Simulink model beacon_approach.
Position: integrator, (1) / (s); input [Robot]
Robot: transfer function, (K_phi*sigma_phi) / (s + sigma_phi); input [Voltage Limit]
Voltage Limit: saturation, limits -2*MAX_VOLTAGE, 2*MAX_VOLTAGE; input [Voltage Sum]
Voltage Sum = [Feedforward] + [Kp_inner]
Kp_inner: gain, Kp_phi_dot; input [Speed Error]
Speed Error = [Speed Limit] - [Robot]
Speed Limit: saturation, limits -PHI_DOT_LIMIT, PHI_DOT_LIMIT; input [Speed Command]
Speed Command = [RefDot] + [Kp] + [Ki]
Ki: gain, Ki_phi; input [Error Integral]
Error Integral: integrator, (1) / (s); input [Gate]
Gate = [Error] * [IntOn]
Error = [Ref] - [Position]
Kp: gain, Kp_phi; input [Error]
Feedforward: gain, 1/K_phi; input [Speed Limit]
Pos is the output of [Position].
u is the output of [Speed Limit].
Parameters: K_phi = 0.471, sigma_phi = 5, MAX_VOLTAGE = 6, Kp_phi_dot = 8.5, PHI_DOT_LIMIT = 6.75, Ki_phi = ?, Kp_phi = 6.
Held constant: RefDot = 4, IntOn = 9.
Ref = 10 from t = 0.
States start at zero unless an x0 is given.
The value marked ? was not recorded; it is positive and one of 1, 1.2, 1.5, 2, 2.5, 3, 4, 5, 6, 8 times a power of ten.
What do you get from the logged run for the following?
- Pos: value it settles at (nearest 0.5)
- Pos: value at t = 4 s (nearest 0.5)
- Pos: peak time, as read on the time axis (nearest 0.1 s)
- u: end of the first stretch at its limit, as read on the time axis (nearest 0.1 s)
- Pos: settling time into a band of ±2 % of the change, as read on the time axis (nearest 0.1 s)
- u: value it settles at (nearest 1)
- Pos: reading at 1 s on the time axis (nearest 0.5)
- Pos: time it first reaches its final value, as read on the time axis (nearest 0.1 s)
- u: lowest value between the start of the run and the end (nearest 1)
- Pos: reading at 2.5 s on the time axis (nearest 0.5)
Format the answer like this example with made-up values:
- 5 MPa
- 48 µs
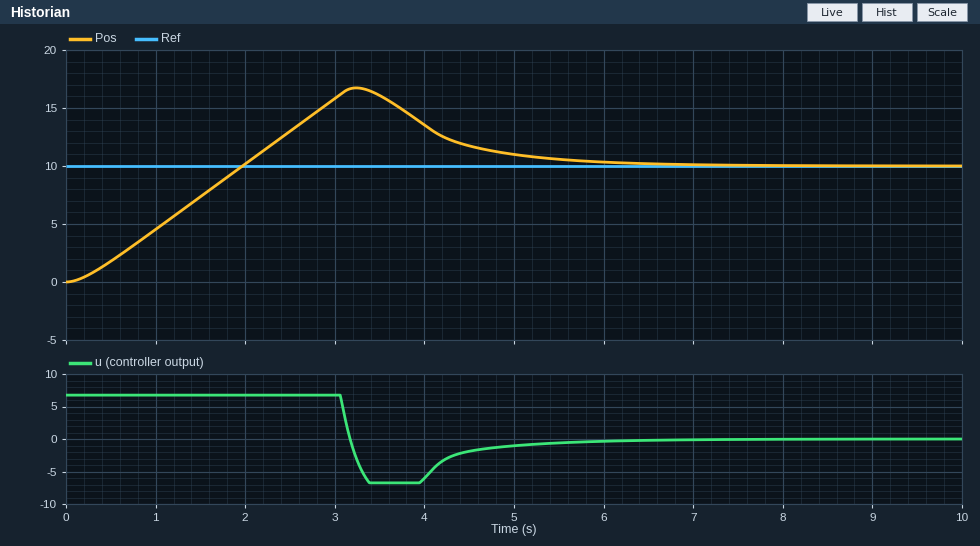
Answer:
- 10.0
- 13.5
- 3.2 s
- 3.1 s
- 6.5 s
- 0
- 4.5
- 2.0 s
- -7
- 13.0
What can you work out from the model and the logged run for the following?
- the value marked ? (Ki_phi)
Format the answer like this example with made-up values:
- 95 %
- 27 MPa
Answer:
- 0.6
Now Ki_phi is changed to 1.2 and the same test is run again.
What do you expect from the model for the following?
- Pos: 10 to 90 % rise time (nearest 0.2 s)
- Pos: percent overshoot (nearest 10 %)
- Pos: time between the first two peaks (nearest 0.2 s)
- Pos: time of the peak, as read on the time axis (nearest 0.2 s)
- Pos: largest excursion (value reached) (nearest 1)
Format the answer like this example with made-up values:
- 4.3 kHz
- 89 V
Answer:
- 1.4 s
- 90 %
- 4.0 s
- 3.6 s
- 19
